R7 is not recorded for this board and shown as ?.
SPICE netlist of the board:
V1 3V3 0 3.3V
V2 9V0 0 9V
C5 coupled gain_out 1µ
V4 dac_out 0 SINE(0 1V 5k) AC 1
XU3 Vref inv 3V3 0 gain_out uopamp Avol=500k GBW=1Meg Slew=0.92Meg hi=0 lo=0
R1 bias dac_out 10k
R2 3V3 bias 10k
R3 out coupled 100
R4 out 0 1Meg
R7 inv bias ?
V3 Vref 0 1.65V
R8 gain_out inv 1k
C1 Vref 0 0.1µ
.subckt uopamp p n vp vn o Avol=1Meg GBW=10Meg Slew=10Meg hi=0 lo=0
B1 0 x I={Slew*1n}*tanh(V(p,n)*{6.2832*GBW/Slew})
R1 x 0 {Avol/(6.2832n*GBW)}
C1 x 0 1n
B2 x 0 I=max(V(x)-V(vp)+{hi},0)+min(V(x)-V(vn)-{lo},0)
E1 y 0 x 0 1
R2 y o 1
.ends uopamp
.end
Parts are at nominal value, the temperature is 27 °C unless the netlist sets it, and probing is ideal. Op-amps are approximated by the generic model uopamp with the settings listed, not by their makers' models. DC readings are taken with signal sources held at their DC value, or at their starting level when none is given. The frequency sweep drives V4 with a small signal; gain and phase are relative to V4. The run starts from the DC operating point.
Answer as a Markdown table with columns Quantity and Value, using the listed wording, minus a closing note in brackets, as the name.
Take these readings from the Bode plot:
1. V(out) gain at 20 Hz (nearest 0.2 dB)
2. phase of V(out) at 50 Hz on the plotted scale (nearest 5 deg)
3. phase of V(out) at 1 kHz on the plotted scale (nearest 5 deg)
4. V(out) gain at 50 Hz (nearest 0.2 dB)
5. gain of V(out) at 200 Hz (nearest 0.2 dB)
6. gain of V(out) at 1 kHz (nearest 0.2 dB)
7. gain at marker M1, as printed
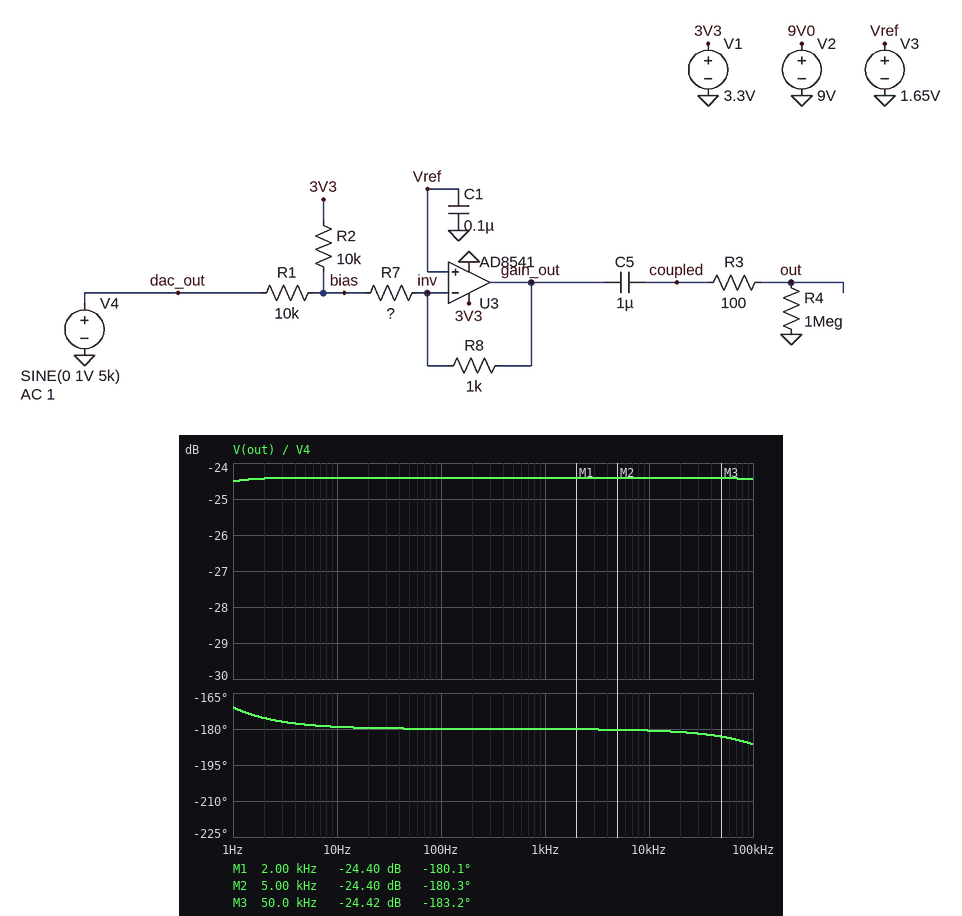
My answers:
| Quantity | Value |
|---|---|
| V(out) gain at 20 Hz | -24.4 dB |
| phase of V(out) at 50 Hz on the plotted scale | -180 deg |
| phase of V(out) at 1 kHz on the plotted scale | -180 deg |
| V(out) gain at 50 Hz | -24.4 dB |
| gain of V(out) at 200 Hz | -24.4 dB |
| gain of V(out) at 1 kHz | -24.4 dB |
| gain at marker M1, as printed | -24.40 dB |
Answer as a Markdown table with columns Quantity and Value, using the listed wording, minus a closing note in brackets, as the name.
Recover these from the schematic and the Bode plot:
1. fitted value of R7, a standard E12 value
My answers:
| Quantity | Value |
|---|---|
| fitted value of R7, a standard E12 value | 3.3 kΩ |
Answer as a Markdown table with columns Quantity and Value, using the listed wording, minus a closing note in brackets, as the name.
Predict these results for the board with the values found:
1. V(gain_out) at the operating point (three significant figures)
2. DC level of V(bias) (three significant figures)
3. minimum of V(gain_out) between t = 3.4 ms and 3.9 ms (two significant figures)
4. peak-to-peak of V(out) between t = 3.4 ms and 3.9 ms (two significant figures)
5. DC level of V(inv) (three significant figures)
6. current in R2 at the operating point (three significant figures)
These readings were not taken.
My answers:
| Quantity | Value |
|---|---|
| V(gain_out) at the operating point | 1.65 V |
| DC level of V(bias) | 1.65 V |
| minimum of V(gain_out) between t = 3.4 ms and 3.9 ms | 1.6 V |
| peak-to-peak of V(out) between t = 3.4 ms and 3.9 ms | 120 mV |
| DC level of V(inv) | 1.65 V |
| current in R2 at the operating point | 165 µA |
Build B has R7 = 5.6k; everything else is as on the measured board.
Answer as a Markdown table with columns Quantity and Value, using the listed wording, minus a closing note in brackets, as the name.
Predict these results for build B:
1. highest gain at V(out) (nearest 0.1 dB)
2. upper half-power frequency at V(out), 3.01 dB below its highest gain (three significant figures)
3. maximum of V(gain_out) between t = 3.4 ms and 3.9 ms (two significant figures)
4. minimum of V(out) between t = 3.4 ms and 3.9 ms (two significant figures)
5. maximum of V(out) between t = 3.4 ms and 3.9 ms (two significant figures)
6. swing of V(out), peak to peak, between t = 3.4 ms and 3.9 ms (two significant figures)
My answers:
| Quantity | Value |
|---|---|
| highest gain at V(out) | -26.5 dB |
| upper half-power frequency at V(out), 3.01 dB below its highest gain | 914 kHz |
| maximum of V(gain_out) between t = 3.4 ms and 3.9 ms | 1.7 V |
| minimum of V(out) between t = 3.4 ms and 3.9 ms | -47 mV |
| maximum of V(out) between t = 3.4 ms and 3.9 ms | 47 mV |
| swing of V(out), peak to peak, between t = 3.4 ms and 3.9 ms | 94 mV |
